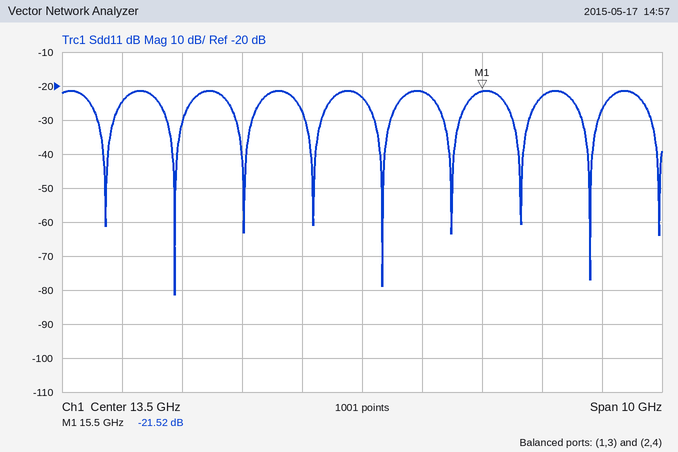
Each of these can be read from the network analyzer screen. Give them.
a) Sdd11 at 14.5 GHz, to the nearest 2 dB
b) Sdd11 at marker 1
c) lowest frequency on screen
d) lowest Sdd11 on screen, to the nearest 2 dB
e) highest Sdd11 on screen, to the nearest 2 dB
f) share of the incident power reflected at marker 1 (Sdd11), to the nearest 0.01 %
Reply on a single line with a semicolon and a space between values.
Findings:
-22 dB; -21.52 dB; 8.5 GHz; -82 dB; -22 dB; 0.70 %
